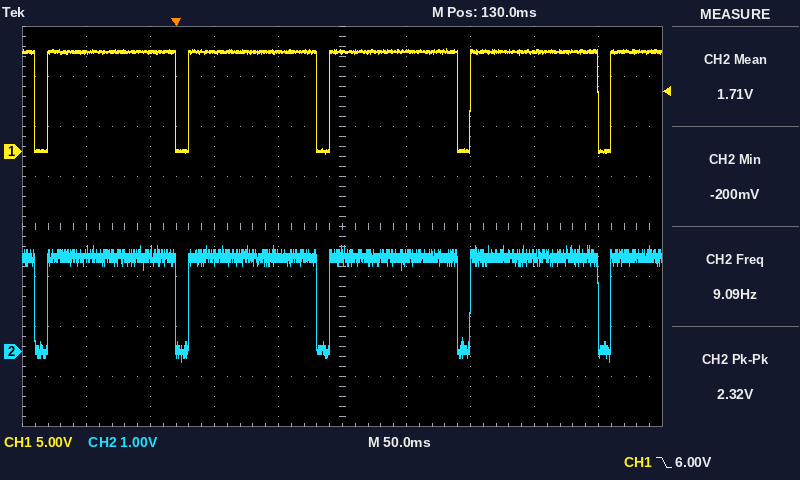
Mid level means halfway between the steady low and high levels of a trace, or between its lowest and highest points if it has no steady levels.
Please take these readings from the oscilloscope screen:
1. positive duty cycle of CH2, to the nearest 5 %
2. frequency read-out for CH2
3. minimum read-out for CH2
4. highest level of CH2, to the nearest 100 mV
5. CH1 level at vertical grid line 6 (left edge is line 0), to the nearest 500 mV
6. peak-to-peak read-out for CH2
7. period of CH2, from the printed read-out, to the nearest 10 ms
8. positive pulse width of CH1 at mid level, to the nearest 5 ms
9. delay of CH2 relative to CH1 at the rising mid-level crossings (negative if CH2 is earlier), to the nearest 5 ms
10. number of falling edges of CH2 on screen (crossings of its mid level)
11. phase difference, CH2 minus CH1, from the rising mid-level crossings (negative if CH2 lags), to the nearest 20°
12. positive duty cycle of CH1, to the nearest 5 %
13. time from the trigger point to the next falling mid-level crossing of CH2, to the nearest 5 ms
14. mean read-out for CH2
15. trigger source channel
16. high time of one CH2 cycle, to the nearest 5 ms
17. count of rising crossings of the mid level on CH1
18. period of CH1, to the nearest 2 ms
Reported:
90 %
9.09 Hz
-200 mV
2.1 V
10.0 V
2.32 V
110 ms
100 ms
0 ms
5
0°
90 %
110 ms
1.71 V
CH1
100 ms
5
110 ms
